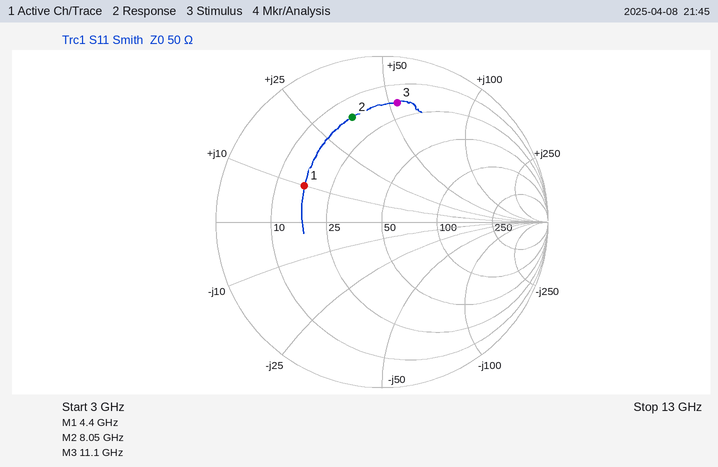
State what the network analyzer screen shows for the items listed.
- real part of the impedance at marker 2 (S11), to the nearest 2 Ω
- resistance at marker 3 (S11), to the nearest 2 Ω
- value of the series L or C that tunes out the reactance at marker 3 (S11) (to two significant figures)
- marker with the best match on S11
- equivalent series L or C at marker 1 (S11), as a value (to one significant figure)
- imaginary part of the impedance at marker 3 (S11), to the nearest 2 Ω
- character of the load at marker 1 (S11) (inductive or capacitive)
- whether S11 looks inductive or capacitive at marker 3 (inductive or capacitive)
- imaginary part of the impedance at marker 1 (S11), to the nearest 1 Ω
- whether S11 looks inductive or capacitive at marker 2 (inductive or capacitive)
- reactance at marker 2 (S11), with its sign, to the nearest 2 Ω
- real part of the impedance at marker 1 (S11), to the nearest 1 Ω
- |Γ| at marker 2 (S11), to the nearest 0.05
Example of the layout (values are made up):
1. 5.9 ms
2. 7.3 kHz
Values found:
1. 16 Ω
2. 18 Ω
3. 270 fF
4. marker 1
5. 400 pH
6. +54 Ω
7. inductive
8. inductive
9. +10 Ω
10. inductive
11. +36 Ω
12. 17 Ω
13. 0.65
